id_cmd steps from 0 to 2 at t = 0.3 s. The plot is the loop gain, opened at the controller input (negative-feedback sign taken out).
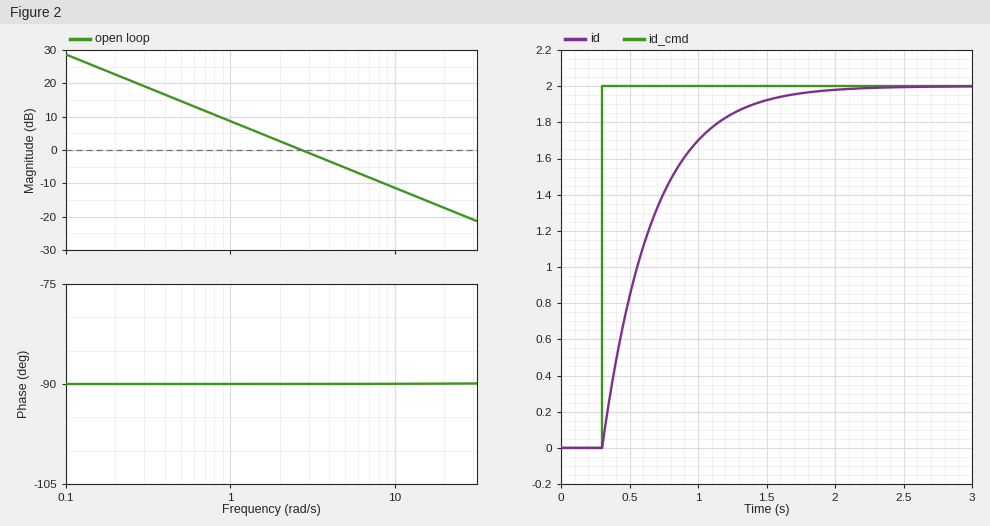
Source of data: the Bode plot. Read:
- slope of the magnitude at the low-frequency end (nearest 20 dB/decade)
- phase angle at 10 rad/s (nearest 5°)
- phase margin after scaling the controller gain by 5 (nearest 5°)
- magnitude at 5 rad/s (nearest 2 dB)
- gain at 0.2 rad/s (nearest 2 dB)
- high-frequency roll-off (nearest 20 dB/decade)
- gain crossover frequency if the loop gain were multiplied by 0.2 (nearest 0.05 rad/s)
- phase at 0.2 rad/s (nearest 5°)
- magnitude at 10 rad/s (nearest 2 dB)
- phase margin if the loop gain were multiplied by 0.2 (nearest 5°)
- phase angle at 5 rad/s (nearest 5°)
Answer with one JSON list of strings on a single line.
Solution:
["-20 dB/decade", "-90°", "90°", "-6 dB", "22 dB", "-20 dB/decade", "0.55 rad/s", "-90°", "-12 dB", "90°", "-90°"]
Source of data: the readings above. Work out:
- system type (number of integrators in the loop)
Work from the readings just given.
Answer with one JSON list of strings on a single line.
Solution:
["1"]
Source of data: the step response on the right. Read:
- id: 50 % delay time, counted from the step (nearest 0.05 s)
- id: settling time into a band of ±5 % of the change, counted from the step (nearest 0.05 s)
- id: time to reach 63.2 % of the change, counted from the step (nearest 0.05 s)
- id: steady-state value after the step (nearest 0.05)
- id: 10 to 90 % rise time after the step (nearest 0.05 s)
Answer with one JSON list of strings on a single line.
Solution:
["0.25 s", "1.10 s", "0.35 s", "2.00", "0.80 s"]
